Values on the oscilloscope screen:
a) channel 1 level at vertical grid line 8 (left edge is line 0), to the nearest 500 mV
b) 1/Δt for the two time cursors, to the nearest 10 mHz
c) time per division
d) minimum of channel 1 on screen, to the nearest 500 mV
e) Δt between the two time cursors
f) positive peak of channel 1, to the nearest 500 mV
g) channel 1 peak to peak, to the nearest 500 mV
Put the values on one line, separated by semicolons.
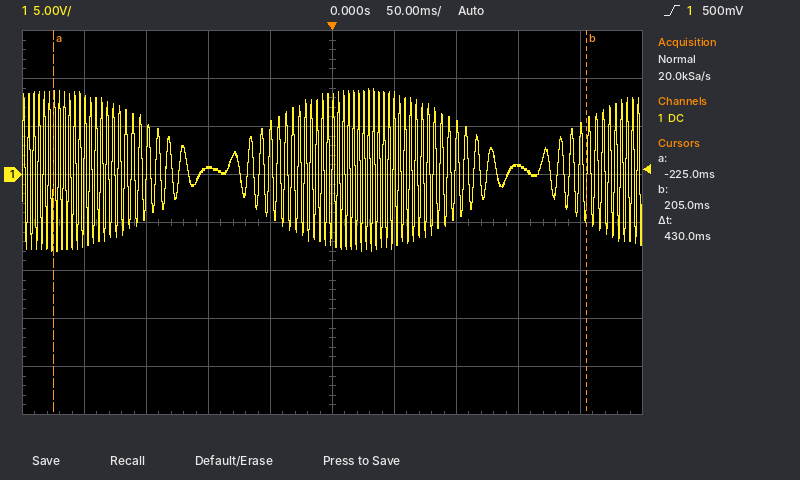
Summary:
1.0 V; 2.33 Hz; 50 ms; -8.0 V; 430 ms; 9.0 V; 17.0 V
